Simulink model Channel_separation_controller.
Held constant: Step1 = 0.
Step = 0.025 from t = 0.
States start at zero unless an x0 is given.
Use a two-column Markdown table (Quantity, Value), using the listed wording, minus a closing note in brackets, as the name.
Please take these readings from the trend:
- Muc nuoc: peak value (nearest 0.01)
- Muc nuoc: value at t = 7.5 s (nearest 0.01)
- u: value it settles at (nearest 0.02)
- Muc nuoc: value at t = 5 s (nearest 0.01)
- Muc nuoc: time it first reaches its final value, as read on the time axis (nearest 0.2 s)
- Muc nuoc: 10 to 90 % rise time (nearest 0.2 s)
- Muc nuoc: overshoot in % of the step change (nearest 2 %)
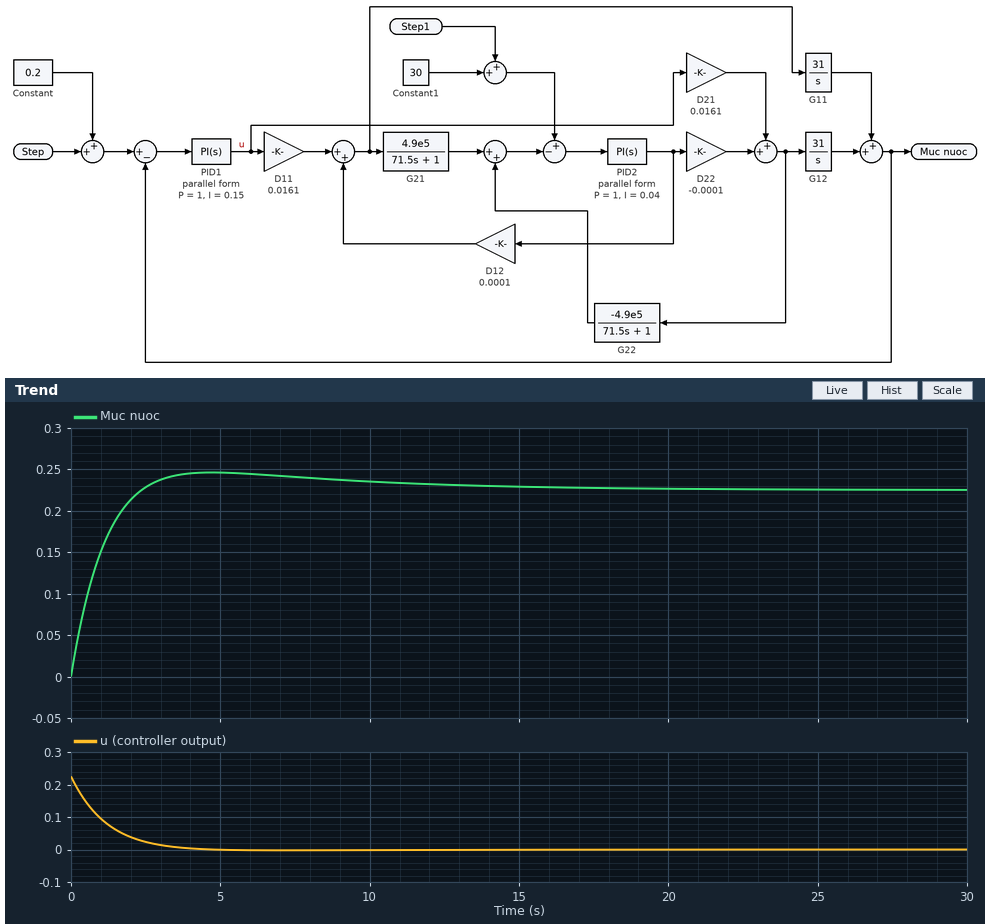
| Quantity | Value |
|---|---|
| Muc nuoc: peak value | 0.25 |
| Muc nuoc: value at t = 7.5 s | 0.24 |
| u: value it settles at | 0.00 |
| Muc nuoc: value at t = 5 s | 0.25 |
| Muc nuoc: time it first reaches its final value, as read on the time axis | 2.4 s |
| Muc nuoc: 10 to 90 % rise time | 1.6 s |
| Muc nuoc: overshoot in % of the step change | 10 % |
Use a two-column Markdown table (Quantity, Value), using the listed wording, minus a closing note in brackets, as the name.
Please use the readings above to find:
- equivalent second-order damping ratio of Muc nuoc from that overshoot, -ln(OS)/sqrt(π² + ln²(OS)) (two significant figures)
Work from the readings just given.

| Quantity | Value |
|---|---|
| equivalent second-order damping ratio of Muc nuoc from that overshoot, -ln(OS)/sqrt(π² + ln²(OS)) | 0.59 |
